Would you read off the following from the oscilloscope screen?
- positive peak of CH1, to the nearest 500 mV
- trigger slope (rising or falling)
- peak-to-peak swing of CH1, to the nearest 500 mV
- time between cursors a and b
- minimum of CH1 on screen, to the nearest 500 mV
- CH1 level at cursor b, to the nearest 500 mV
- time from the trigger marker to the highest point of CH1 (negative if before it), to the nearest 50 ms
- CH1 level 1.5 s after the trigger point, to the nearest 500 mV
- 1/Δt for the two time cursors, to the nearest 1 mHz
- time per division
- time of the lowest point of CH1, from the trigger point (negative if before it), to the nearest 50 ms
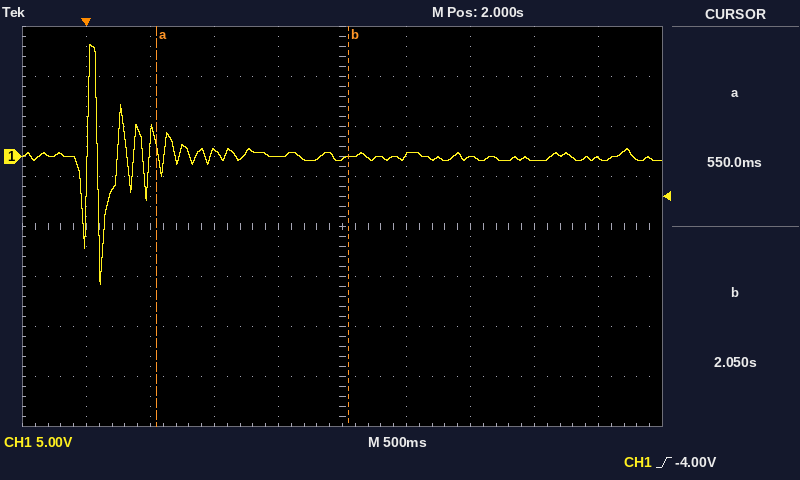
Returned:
11.0 V
rising
24.0 V
1.50 s
-13.0 V
0.0 V
+50 ms
0.0 V
667 mHz
500 ms
+100 ms
